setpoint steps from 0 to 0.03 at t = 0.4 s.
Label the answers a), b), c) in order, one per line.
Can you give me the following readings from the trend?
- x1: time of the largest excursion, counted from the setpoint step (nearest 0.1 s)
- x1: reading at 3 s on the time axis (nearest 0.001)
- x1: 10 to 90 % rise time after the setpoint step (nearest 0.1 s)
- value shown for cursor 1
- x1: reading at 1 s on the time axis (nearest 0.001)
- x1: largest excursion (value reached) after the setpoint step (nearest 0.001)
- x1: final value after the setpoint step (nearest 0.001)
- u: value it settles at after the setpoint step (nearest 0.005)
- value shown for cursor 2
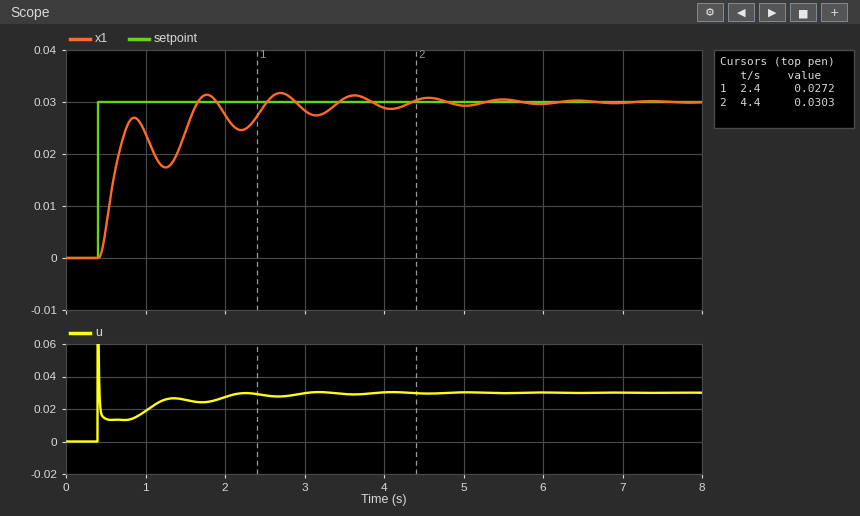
a) 2.3 s
b) 0.028
c) 1.1 s
d) 0.0272
e) 0.024
f) 0.032
g) 0.030
h) 0.030
i) 0.0303
